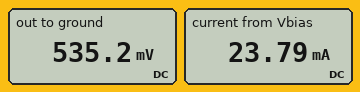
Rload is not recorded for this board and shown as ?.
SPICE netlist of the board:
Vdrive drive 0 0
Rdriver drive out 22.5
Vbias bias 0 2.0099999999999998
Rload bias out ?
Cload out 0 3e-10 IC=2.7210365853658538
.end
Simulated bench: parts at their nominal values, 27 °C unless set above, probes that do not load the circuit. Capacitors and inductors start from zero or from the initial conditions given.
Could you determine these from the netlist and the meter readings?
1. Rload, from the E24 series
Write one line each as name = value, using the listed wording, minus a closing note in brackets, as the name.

Rload, from the E24 series = 62 Ω
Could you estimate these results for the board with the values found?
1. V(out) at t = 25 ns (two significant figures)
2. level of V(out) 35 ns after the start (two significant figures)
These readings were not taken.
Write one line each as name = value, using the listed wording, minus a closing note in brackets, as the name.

V(out) at t = 25 ns = 550 mV
level of V(out) 35 ns after the start = 540 mV
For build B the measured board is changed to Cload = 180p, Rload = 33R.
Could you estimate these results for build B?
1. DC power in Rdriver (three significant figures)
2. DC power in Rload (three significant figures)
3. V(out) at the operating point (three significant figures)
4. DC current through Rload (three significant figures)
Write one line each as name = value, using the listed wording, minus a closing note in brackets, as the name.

DC power in Rdriver = 29.5 mW
DC power in Rload = 43.3 mW
V(out) at the operating point = 815 mV
DC current through Rload = 36.2 mA
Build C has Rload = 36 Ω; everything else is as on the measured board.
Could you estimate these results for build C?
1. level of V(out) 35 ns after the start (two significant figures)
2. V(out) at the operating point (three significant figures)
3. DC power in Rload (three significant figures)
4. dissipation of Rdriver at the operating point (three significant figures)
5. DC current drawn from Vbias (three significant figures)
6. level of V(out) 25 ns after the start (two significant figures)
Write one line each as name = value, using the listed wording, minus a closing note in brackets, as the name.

level of V(out) 35 ns after the start = 770 mV
V(out) at the operating point = 773 mV
DC power in Rload = 42.5 mW
dissipation of Rdriver at the operating point = 26.6 mW
DC current drawn from Vbias = 34.4 mA
level of V(out) 25 ns after the start = 780 mV
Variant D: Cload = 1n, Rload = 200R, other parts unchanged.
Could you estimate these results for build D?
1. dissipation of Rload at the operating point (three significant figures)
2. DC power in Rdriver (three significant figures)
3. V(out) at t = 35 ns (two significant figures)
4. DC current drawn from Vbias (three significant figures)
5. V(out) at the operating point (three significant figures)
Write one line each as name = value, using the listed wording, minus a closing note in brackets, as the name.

dissipation of Rload at the operating point = 16.3 mW
DC power in Rdriver = 1.84 mW
V(out) at t = 35 ns = 650 mV
DC current drawn from Vbias = 9.03 mA
V(out) at the operating point = 203 mV
